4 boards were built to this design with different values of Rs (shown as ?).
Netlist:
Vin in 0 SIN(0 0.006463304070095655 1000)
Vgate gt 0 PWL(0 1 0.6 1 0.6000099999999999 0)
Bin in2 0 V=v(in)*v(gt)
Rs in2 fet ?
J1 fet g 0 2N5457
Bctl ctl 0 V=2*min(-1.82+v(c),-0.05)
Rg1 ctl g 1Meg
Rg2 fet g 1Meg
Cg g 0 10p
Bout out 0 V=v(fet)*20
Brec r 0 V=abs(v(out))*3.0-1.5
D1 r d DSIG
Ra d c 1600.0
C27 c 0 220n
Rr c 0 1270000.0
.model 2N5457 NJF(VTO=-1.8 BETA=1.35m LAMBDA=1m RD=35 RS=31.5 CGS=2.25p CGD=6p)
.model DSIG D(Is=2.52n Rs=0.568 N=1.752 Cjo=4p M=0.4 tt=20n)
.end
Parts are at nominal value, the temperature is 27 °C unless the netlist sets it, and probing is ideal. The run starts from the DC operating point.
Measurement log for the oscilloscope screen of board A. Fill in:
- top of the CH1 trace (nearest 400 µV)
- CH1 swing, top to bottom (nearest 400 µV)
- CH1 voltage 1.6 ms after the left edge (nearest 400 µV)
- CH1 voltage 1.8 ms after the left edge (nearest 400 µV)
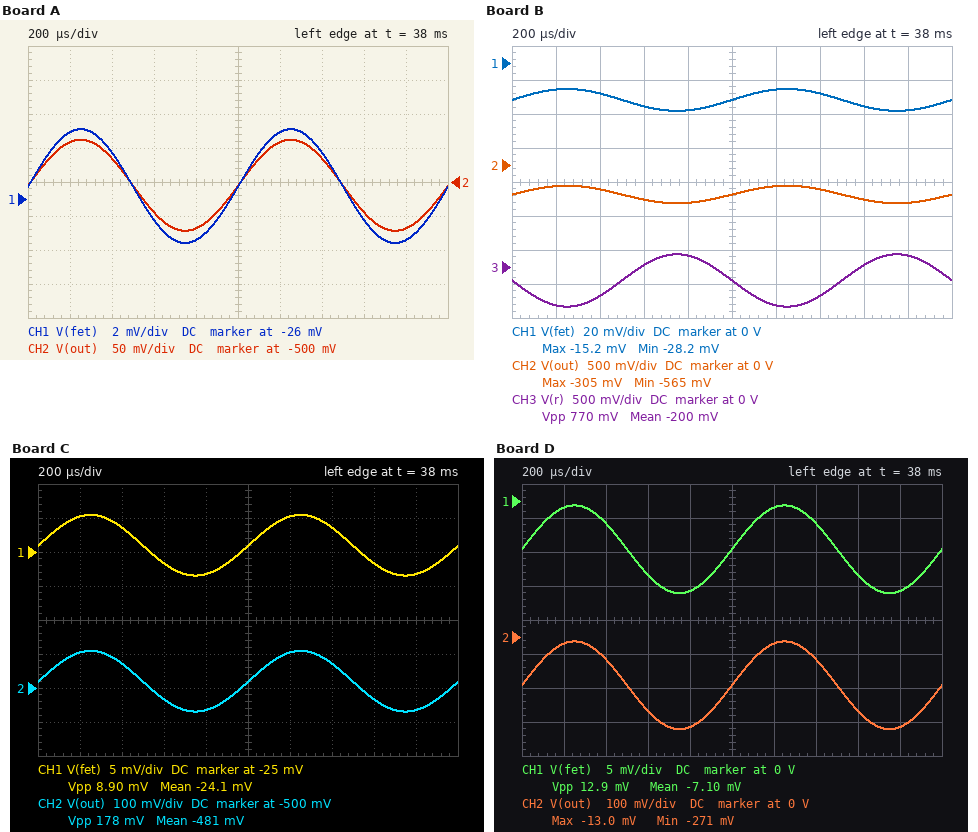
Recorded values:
-22.0 mV
6.8 mV
-27.2 mV
-28.4 mV
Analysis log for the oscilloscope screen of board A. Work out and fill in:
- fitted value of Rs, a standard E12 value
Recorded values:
27 kΩ
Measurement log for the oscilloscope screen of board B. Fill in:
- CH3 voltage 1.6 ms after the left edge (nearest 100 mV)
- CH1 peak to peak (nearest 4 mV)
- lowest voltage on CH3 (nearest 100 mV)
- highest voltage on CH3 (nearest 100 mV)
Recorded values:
0 V
12 mV
-600 mV
200 mV
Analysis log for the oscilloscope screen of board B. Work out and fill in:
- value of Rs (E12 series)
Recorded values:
12 kΩ
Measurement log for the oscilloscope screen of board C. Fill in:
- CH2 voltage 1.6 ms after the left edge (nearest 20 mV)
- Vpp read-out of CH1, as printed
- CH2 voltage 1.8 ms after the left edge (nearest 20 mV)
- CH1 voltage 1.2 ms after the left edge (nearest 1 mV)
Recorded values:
-540 mV
8.90 mV
-560 mV
-20 mV
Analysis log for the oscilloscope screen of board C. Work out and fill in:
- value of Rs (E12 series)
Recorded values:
18 kΩ
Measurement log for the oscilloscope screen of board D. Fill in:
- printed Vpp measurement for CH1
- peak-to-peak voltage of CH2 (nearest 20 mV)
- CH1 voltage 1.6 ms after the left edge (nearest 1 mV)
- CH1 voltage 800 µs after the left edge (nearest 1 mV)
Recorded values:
12.9 mV
260 mV
-11 mV
-13 mV
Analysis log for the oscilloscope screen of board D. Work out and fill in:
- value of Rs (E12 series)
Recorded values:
3.9 kΩ
